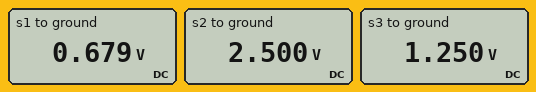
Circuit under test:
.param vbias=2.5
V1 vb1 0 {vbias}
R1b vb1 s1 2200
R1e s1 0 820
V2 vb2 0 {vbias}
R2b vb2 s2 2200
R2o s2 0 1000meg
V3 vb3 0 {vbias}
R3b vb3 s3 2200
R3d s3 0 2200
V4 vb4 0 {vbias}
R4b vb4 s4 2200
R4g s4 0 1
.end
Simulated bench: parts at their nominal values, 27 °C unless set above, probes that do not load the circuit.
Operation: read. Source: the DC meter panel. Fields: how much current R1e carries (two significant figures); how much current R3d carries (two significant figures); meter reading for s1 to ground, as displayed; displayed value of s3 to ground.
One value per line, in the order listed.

830 µA
570 µA
0.679 V
1.250 V
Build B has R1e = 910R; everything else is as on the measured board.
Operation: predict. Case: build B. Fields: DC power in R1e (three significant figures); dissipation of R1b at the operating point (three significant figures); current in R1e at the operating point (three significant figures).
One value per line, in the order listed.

588 µW
1.42 mW
804 µA
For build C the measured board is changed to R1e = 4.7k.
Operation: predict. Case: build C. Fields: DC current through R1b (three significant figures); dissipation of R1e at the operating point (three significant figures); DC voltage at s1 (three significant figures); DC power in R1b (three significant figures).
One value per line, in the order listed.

362 µA
617 µW
1.70 V
289 µW
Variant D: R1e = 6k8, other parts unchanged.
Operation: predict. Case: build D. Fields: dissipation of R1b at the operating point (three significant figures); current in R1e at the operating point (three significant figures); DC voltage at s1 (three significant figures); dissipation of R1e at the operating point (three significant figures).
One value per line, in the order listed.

170 µW
278 µA
1.89 V
525 µW
